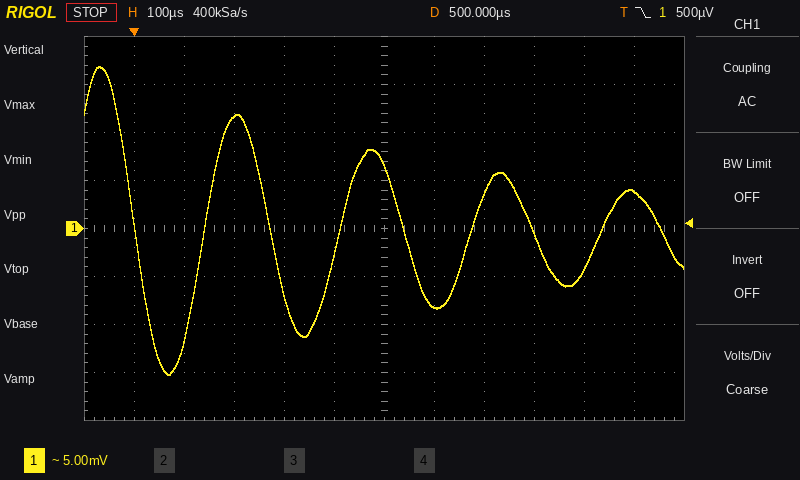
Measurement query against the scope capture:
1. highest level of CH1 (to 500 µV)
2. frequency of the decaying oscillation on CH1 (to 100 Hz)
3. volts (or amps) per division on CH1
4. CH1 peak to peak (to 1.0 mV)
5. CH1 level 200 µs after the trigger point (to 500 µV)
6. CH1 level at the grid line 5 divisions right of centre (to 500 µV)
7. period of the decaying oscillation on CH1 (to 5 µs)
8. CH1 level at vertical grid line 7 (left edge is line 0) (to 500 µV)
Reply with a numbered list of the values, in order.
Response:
1. 17.0 mV
2. 3.8 kHz
3. 5 mV
4. 32.0 mV
5. 11.5 mV
6. 4.0 mV
7. 265 µs
8. -8.0 mV
